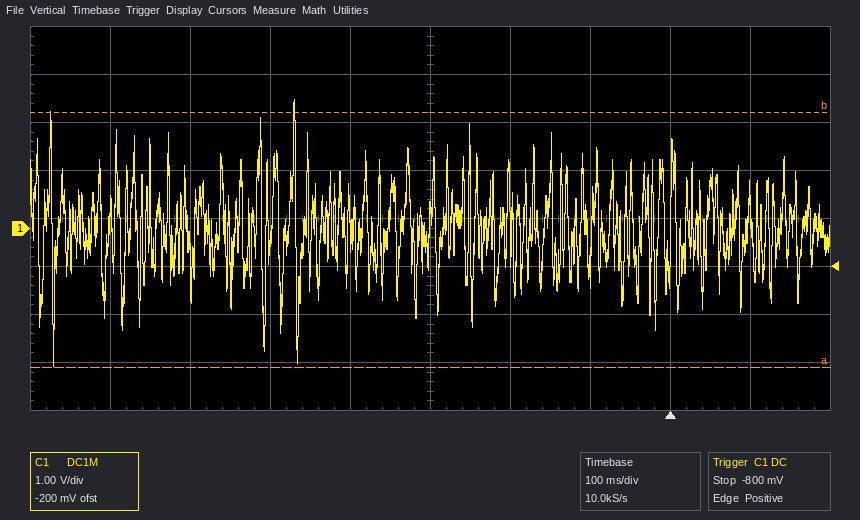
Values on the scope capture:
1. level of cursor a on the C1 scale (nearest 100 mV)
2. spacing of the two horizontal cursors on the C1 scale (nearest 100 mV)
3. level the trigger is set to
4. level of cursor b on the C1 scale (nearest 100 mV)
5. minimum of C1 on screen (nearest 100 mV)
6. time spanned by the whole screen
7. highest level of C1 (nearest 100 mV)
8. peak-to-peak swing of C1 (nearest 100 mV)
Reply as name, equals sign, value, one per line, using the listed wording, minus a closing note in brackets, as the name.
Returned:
level of cursor a on the C1 scale = -2.9 V
spacing of the two horizontal cursors on the C1 scale = 5.3 V
level the trigger is set to = -800 mV
level of cursor b on the C1 scale = 2.4 V
minimum of C1 on screen = -2.9 V
time spanned by the whole screen = 1 s
highest level of C1 = 2.7 V
peak-to-peak swing of C1 = 5.6 V
